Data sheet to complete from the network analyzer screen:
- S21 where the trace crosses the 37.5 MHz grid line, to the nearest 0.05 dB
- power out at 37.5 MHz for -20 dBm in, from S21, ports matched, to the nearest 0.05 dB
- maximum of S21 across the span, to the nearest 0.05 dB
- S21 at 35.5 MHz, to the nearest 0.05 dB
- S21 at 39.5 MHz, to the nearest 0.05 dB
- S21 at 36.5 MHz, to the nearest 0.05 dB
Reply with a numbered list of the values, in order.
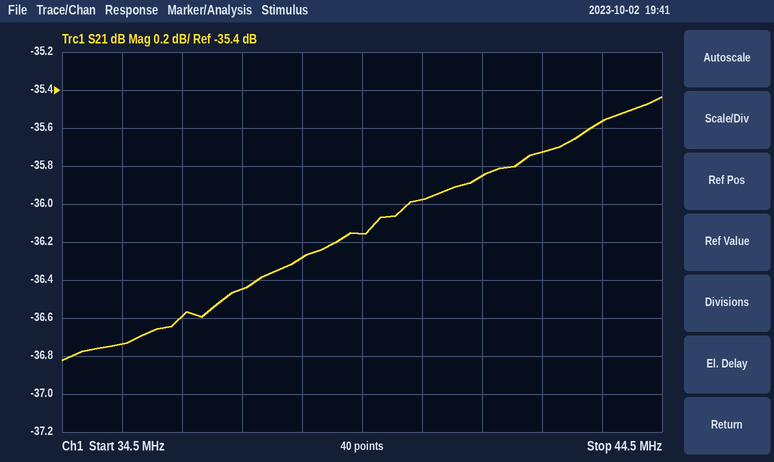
1. -36.45 dB
2. -56.45 dBm
3. -35.45 dB
4. -36.75 dB
5. -36.15 dB
6. -36.60 dB
